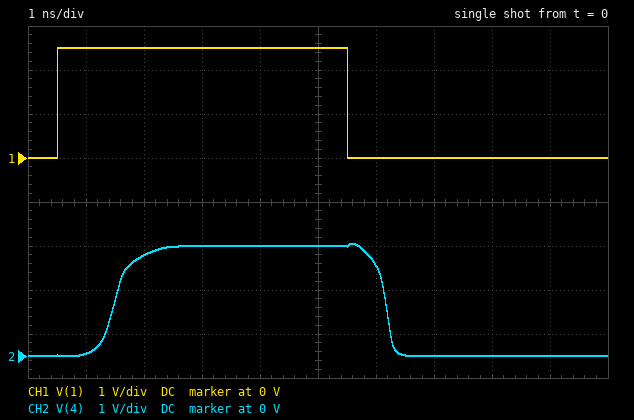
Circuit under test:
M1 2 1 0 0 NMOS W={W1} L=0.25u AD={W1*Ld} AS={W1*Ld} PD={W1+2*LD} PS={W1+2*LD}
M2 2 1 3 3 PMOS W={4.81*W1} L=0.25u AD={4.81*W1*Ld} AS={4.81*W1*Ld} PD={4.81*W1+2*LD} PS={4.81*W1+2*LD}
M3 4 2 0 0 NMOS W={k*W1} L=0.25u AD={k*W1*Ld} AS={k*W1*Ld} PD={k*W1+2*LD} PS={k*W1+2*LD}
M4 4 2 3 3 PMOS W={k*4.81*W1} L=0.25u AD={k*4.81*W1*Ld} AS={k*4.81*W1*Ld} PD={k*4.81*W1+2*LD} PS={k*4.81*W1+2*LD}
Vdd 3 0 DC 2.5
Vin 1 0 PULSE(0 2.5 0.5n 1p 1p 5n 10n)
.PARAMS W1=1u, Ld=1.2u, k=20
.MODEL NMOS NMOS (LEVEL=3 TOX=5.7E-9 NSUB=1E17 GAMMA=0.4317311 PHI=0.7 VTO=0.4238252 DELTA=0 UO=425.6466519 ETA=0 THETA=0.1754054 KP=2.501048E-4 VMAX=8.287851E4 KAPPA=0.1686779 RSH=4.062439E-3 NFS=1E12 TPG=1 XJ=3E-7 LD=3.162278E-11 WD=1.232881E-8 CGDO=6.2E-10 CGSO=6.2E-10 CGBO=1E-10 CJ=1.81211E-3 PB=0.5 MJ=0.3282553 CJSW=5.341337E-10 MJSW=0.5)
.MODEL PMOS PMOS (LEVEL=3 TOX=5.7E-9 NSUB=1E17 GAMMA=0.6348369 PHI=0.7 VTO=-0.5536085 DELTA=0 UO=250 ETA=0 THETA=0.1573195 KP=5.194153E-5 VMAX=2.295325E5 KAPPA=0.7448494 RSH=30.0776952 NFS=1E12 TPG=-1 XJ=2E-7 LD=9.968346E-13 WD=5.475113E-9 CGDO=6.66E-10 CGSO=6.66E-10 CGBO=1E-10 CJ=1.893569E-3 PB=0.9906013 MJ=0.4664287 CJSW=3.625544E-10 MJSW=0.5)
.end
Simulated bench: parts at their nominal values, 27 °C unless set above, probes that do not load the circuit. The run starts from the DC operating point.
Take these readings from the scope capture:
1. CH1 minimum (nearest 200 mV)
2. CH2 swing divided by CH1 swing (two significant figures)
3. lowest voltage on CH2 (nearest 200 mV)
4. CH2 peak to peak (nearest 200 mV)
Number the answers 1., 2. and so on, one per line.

1. 0 V
2. 1.0
3. 0 V
4. 2.6 V
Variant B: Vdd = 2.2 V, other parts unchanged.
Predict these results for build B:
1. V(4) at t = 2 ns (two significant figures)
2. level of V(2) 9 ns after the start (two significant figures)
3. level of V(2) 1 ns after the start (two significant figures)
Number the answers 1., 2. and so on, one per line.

1. 2.1 V
2. 2.2 V
3. 1.4 V
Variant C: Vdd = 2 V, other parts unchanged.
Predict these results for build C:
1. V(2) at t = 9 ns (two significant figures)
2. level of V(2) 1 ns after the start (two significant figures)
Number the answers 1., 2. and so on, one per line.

1. 2.0 V
2. 1.2 V
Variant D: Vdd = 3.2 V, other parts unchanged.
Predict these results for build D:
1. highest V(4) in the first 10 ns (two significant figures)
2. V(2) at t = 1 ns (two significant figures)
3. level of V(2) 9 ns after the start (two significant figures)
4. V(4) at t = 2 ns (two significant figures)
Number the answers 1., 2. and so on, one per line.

1. 3.3 V
2. 2.4 V
3. 3.2 V
4. 2.5 V
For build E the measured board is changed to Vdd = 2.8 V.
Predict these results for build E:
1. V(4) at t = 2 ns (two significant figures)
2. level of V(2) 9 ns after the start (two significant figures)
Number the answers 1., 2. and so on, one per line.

1. 2.4 V
2. 2.8 V
